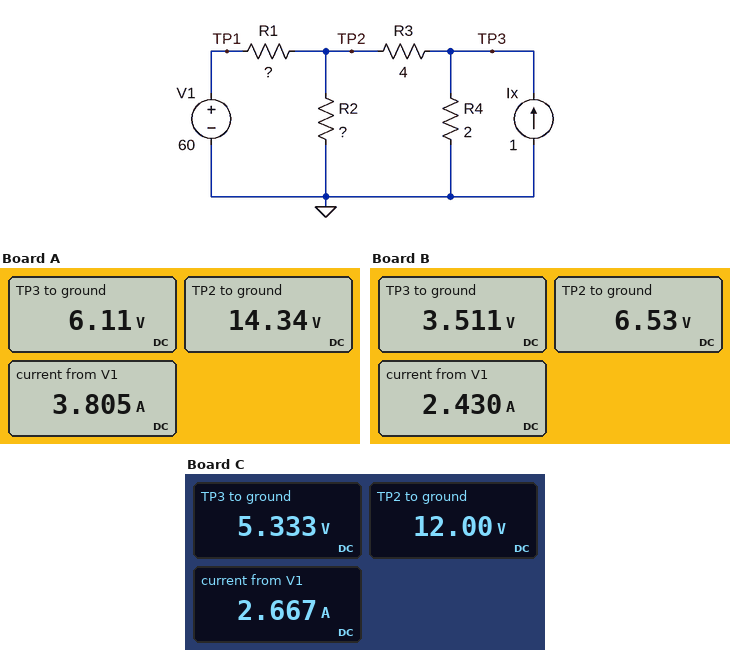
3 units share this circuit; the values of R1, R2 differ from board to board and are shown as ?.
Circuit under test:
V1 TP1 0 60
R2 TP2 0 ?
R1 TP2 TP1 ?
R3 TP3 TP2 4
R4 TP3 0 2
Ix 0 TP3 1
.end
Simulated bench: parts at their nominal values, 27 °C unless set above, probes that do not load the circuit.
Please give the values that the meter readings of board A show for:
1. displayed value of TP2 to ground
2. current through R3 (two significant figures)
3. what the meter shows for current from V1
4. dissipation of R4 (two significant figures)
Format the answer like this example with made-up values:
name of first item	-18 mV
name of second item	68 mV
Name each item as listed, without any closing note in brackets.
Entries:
displayed value of TP2 to ground	14.34 V
current through R3	2.1 A
what the meter shows for current from V1	3.805 A
dissipation of R4	19 W
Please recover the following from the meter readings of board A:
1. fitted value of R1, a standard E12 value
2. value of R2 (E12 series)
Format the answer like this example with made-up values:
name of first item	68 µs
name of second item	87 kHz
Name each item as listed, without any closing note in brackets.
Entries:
fitted value of R1, a standard E12 value	12 Ω
value of R2	8.2 Ω
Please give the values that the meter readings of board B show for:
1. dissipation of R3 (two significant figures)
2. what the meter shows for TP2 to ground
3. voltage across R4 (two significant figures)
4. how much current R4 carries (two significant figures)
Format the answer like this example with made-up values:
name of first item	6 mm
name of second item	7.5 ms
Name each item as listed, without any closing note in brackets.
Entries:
dissipation of R3	2.3 W
what the meter shows for TP2 to ground	6.53 V
voltage across R4	3.5 V
how much current R4 carries	1.8 A
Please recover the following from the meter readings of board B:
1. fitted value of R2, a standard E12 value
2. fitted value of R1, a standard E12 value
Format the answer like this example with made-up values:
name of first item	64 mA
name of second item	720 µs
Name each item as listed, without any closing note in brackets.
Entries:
fitted value of R2, a standard E12 value	3.9 Ω
fitted value of R1, a standard E12 value	22 Ω
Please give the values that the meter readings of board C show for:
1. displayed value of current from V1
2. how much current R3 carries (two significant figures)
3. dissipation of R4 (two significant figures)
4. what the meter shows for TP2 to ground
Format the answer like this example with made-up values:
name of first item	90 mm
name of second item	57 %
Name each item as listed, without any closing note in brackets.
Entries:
displayed value of current from V1	2.667 A
how much current R3 carries	1.7 A
dissipation of R4	14 W
what the meter shows for TP2 to ground	12.00 V
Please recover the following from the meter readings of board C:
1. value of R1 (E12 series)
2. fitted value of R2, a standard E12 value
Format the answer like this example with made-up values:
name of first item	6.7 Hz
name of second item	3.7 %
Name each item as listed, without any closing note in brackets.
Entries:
value of R1	18 Ω
fitted value of R2, a standard E12 value	12 Ω
